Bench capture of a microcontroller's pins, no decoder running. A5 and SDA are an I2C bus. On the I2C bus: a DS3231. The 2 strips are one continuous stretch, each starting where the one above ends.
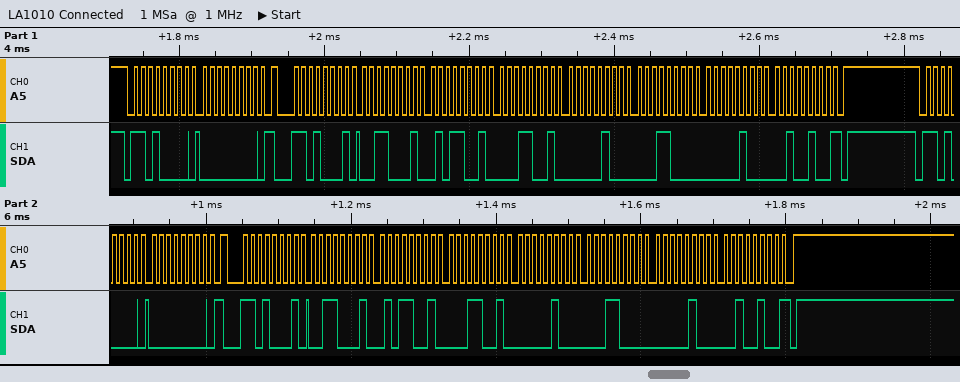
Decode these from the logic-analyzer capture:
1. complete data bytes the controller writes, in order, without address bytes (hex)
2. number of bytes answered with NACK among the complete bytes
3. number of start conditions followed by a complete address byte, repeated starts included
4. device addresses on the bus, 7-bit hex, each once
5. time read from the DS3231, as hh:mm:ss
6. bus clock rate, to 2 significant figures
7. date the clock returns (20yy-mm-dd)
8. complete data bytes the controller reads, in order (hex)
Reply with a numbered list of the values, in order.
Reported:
1. 00 00
2. 2
3. 4
4. 0x68
5. 19:59:31
6. 100 kHz
7. 2024-04-18
8. 31 59 19 04 18 04 24 31 59 19 04 18 04 24
